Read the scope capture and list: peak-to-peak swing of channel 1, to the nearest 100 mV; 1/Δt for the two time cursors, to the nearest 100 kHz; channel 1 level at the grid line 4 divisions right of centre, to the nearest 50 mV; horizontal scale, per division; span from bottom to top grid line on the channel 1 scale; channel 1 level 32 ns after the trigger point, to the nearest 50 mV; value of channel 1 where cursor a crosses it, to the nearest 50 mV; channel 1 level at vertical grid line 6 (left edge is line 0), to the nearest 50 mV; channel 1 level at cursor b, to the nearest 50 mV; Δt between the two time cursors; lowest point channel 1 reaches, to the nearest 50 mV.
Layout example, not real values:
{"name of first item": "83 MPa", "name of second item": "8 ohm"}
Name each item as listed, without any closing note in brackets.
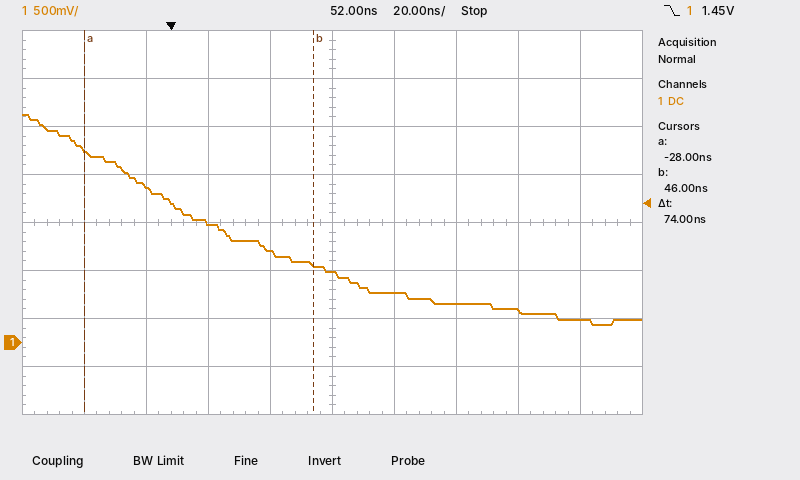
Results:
{"peak-to-peak swing of channel 1, to the nearest 100 mV": "2.20 V", "1/Δt for the two time cursors, to the nearest 100 kHz": "13.5 MHz", "channel 1 level at the grid line 4 divisions right of centre, to the nearest 50 mV": "250 mV", "horizontal scale, per division": "20 ns", "span from bottom to top grid line on the channel 1 scale": "4 V", "channel 1 level 32 ns after the trigger point, to the nearest 50 mV": "950 mV", "value of channel 1 where cursor a crosses it, to the nearest 50 mV": "2.00 V", "channel 1 level at vertical grid line 6 (left edge is line 0), to the nearest 50 mV": "500 mV", "channel 1 level at cursor b, to the nearest 50 mV": "800 mV", "Δt between the two time cursors": "74 ns", "lowest point channel 1 reaches, to the nearest 50 mV": "200 mV"}
